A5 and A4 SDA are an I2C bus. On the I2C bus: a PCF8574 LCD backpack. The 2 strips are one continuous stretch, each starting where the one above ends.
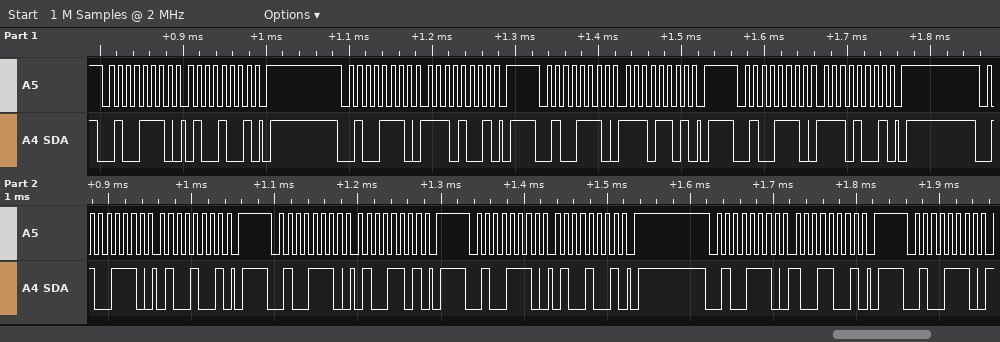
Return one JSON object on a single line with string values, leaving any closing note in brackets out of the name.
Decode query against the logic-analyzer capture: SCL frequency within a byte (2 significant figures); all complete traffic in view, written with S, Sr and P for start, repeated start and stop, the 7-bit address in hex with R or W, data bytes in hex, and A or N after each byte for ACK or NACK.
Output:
{"SCL frequency within a byte": "100 kHz", "all complete traffic in view, written with S, Sr and P for start, repeated start and stop, the 7-bit address in hex with R or W, data bytes in hex, and A or N after each byte for ACK or NACK": "S 27W A 49 A P S 27W A E9 A P S 27W A ED A P S 27W A E9 A P S 27W A 49 A P S 27W A 4D A P S 27W A 49 A P S 27W A 99 A P S 27W A"}
